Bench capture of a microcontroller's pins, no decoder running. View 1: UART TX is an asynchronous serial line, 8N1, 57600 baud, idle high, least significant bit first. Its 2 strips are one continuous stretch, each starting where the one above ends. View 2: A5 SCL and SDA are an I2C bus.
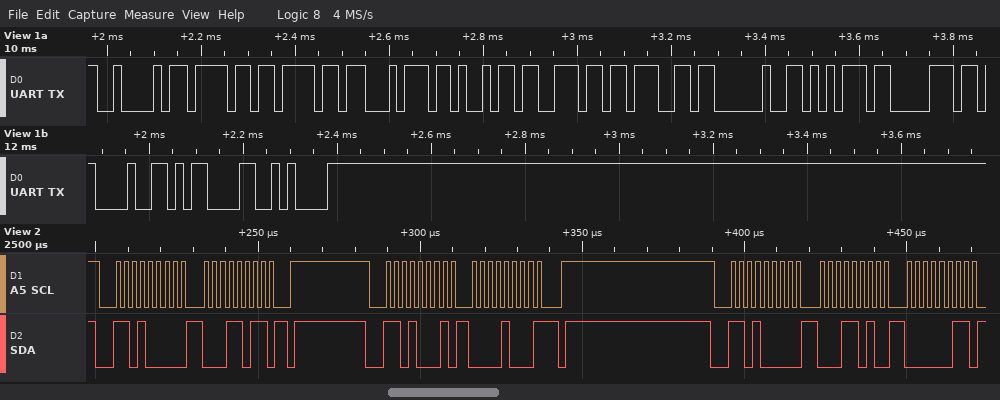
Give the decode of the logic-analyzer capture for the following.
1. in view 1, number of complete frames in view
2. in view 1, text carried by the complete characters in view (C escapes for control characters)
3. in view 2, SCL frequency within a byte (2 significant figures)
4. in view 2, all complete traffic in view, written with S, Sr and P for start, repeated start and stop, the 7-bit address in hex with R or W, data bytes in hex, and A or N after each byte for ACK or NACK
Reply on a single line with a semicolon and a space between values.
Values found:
13; "Booting up!\r\n"; 400 kHz; S 68W A 1B A P S 68R A 08 N P S 68W A 1A A 03 A
